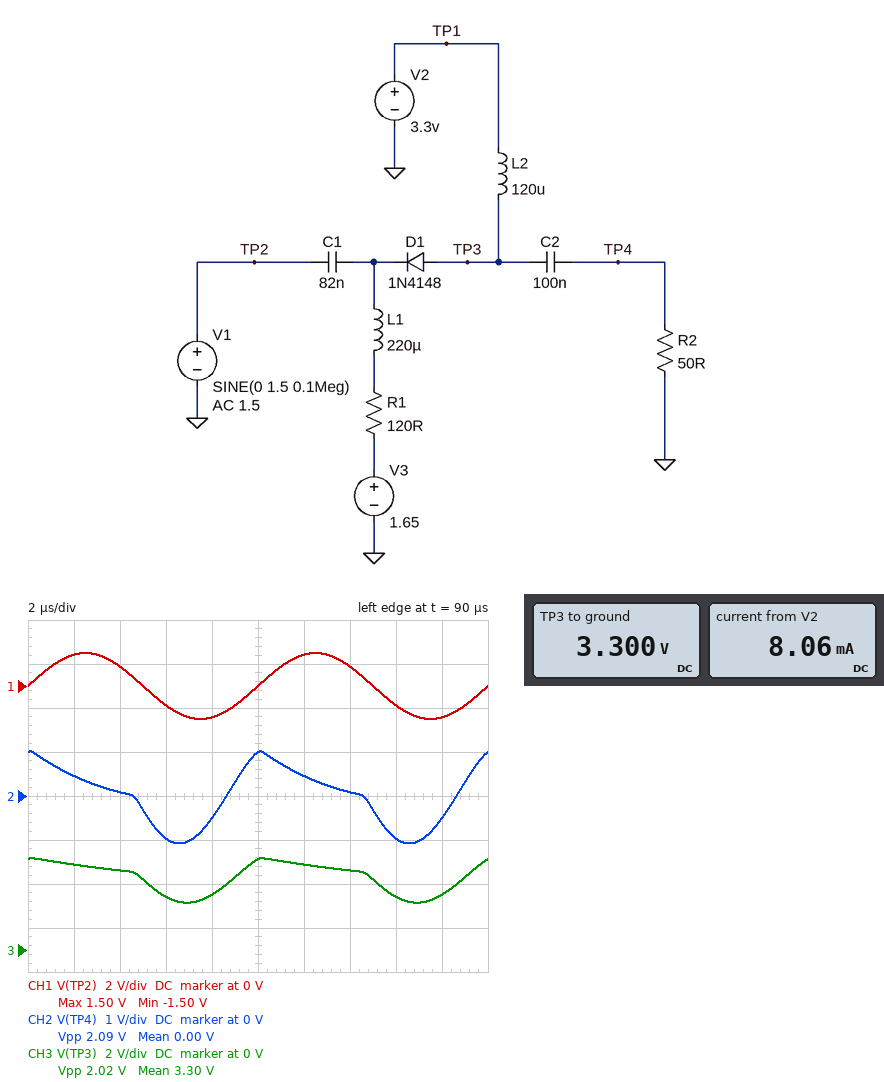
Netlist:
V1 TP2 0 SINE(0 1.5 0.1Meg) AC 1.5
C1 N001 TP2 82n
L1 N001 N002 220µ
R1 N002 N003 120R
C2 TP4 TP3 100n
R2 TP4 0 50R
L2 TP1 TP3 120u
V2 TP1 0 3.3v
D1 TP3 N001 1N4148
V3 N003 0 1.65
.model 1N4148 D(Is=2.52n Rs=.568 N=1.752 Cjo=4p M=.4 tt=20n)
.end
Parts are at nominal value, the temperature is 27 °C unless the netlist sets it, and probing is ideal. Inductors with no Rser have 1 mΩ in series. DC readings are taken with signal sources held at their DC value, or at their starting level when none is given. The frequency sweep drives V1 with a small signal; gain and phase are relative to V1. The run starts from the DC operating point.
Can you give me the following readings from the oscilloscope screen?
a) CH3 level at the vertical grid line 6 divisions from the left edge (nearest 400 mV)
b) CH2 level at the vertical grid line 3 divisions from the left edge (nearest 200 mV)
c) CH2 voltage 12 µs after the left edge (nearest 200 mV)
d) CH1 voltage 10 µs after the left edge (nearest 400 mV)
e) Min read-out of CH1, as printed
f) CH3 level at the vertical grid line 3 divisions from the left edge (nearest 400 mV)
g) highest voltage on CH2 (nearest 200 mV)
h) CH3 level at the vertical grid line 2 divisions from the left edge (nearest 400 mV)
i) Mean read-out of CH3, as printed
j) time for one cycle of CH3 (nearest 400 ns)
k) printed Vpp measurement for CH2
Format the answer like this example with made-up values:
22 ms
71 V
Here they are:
4.0 V
-1.0 V
400 mV
0 V
-1.50 V
2.4 V
1.0 V
3.6 V
3.30 V
10.0 µs
2.09 V
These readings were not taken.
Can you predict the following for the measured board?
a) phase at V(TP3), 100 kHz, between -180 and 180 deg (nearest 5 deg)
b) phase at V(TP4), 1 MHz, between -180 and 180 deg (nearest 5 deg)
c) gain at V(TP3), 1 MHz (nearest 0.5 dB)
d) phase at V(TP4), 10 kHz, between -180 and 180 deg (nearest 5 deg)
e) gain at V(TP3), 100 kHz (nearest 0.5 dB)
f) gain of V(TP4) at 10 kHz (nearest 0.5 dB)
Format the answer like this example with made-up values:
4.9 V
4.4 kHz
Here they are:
30 deg
5 deg
-1.0 dB
-115 deg
0 dB
-38.5 dB
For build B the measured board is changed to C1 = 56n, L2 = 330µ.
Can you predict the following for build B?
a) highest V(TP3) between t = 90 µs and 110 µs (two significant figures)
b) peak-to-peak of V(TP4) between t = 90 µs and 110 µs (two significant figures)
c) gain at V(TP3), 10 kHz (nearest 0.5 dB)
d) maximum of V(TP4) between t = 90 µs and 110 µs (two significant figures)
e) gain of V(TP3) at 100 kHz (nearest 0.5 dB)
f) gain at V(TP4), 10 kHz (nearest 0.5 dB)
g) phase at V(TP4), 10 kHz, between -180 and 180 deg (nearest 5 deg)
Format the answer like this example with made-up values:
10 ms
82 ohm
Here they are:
3.9 V
1.8 V
-22.0 dB
720 mV
-1.5 dB
-32.5 dB
-120 deg
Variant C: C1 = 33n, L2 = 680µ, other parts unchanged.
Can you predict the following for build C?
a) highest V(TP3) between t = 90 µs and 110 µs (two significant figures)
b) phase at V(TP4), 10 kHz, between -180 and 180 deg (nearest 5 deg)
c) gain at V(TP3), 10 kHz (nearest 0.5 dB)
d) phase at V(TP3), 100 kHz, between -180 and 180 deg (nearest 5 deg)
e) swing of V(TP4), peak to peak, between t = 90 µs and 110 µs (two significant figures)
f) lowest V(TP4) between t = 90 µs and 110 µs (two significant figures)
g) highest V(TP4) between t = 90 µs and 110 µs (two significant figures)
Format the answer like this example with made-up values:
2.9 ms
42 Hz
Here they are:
4.0 V
-140 deg
-20.0 dB
45 deg
1.5 V
-920 mV
590 mV
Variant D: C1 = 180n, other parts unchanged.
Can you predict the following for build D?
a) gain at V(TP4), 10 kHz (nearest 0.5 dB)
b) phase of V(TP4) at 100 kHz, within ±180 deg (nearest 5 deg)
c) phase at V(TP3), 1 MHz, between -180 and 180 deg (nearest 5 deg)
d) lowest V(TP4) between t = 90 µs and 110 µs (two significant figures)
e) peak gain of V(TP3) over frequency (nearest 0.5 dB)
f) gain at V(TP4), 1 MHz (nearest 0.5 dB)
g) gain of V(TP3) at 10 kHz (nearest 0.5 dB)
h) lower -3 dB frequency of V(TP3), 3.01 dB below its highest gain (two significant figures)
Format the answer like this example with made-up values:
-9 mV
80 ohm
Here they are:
-31.5 dB
30 deg
0 deg
-1.0 V
3.5 dB
-1.0 dB
-21.0 dB
26 kHz
